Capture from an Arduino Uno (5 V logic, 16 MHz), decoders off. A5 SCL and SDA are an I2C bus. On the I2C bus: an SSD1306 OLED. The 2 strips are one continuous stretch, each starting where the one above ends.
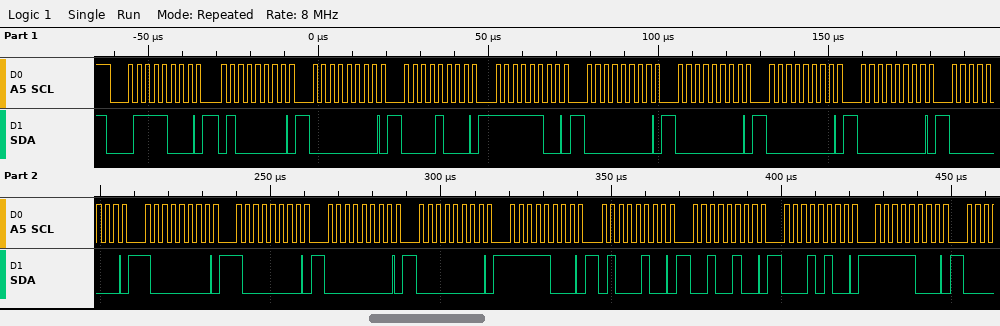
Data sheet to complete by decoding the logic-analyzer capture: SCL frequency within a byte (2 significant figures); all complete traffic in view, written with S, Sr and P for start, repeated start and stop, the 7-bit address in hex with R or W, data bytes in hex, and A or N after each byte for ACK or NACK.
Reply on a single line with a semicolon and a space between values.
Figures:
400 kHz; S 3CW A 40 A 00 A 08 A FC A 00 A 00 A 00 A 00 A 00 A 80 A 80 A 00 A 00 A F8 A 44 A 24 A 14 A F8 A
